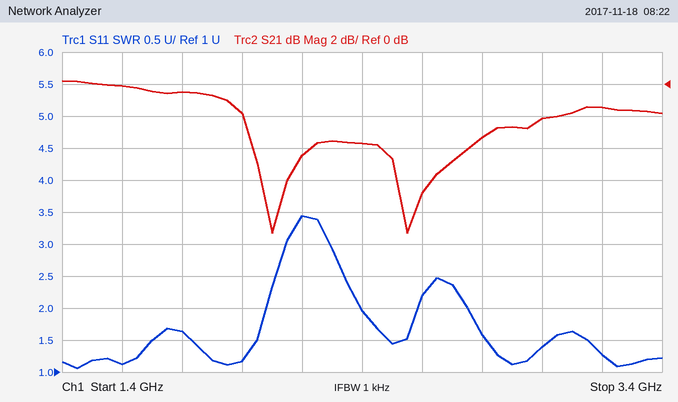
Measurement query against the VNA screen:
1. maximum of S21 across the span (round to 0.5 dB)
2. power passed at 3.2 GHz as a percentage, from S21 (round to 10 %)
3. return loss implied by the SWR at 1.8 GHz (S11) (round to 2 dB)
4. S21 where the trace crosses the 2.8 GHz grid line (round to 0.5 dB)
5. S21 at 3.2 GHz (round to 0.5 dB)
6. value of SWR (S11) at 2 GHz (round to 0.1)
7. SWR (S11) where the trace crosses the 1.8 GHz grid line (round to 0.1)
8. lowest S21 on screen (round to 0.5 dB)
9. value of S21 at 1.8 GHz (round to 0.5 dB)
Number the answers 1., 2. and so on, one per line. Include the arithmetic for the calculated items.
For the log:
1. 0.0 dB
2. 10^(-1.5/10) ≈ 70.8 %, so 70 % to the nearest 10 %
3. −20 log10((1.6 − 1)/(1.6 + 1)) ≈ 12.7 dB, so 12 dB to the nearest 2 dB
4. -3.5 dB
5. -1.5 dB
6. 1.2
7. 1.6
8. -9.5 dB
9. -0.5 dB
